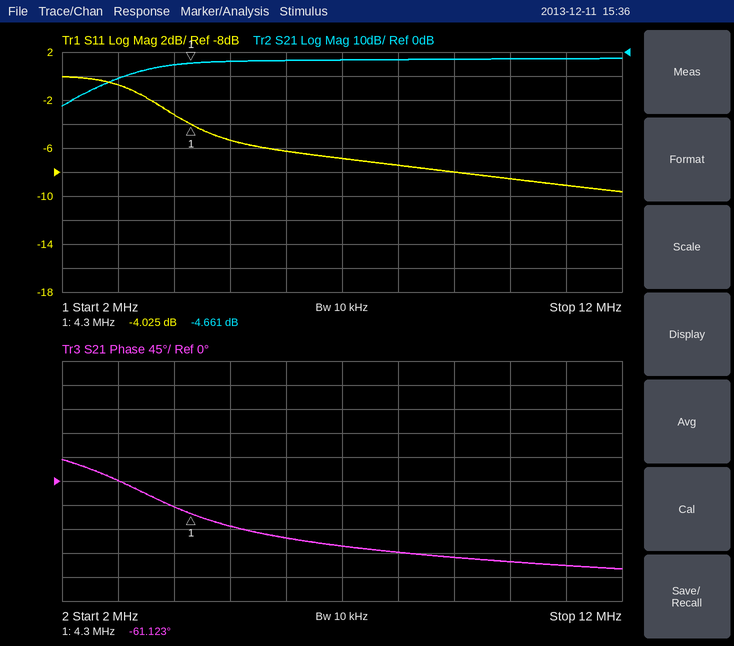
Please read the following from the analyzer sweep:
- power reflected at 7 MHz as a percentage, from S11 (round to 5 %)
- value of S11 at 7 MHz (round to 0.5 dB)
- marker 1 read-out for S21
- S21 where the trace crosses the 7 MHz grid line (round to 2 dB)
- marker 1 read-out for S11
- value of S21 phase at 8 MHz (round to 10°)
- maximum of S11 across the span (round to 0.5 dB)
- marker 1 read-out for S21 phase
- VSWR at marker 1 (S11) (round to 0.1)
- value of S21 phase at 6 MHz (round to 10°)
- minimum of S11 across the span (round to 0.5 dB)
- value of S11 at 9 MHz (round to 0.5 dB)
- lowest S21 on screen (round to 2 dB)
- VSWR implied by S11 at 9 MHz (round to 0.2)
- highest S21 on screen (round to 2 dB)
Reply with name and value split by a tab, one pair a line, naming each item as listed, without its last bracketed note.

power reflected at 7 MHz as a percentage, from S11	20 %
value of S11 at 7 MHz	-7.0 dB
marker 1 read-out for S21	-4.661 dB
S21 where the trace crosses the 7 MHz grid line	-4 dB
marker 1 read-out for S11	-4.025 dB
value of S21 phase at 8 MHz	-130°
maximum of S11 across the span	0.0 dB
marker 1 read-out for S21 phase	-61.123°
VSWR at marker 1 (S11)	4.4
value of S21 phase at 6 MHz	-110°
minimum of S11 across the span	-9.5 dB
value of S11 at 9 MHz	-8.0 dB
lowest S21 on screen	-22 dB
VSWR implied by S11 at 9 MHz	2.4
highest S21 on screen	-2 dB
